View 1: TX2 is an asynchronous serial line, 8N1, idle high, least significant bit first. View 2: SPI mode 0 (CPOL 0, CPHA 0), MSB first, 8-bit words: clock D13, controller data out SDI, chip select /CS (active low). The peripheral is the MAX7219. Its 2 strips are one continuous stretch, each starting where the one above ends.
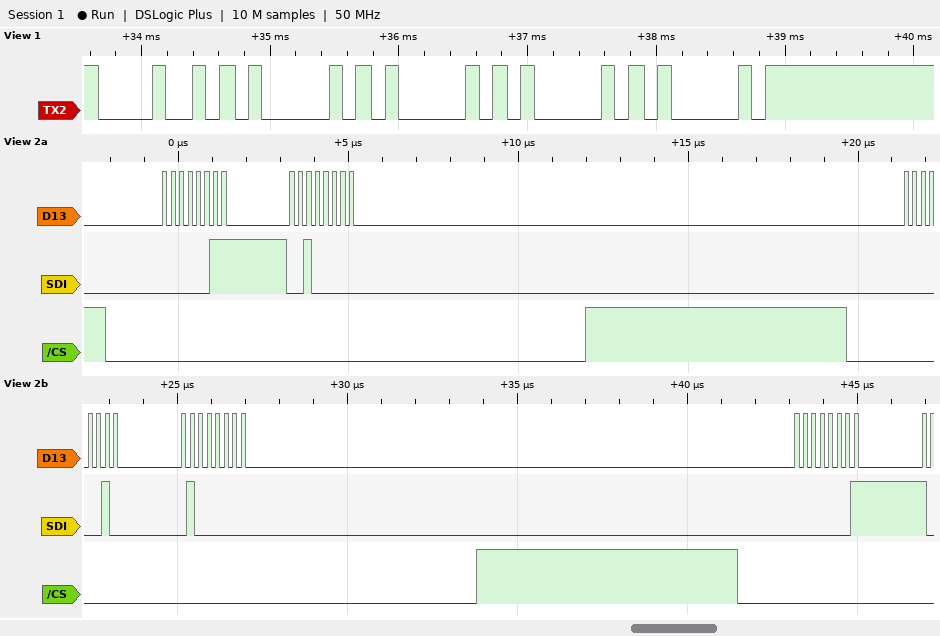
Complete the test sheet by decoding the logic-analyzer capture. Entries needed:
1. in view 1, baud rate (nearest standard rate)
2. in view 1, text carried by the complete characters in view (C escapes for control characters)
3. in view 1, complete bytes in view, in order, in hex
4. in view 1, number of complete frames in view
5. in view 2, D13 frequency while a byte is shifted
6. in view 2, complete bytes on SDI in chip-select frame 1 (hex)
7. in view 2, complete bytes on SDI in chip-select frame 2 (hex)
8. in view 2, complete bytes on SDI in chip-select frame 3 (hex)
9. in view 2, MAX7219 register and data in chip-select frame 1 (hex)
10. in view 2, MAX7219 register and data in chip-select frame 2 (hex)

9600 baud
"HAAAA"
48 41 41 41 41
5
4 MHz
0x03 0x20
0x02 0x40
0x01
register 0x3, data 0x20
register 0x2, data 0x40
